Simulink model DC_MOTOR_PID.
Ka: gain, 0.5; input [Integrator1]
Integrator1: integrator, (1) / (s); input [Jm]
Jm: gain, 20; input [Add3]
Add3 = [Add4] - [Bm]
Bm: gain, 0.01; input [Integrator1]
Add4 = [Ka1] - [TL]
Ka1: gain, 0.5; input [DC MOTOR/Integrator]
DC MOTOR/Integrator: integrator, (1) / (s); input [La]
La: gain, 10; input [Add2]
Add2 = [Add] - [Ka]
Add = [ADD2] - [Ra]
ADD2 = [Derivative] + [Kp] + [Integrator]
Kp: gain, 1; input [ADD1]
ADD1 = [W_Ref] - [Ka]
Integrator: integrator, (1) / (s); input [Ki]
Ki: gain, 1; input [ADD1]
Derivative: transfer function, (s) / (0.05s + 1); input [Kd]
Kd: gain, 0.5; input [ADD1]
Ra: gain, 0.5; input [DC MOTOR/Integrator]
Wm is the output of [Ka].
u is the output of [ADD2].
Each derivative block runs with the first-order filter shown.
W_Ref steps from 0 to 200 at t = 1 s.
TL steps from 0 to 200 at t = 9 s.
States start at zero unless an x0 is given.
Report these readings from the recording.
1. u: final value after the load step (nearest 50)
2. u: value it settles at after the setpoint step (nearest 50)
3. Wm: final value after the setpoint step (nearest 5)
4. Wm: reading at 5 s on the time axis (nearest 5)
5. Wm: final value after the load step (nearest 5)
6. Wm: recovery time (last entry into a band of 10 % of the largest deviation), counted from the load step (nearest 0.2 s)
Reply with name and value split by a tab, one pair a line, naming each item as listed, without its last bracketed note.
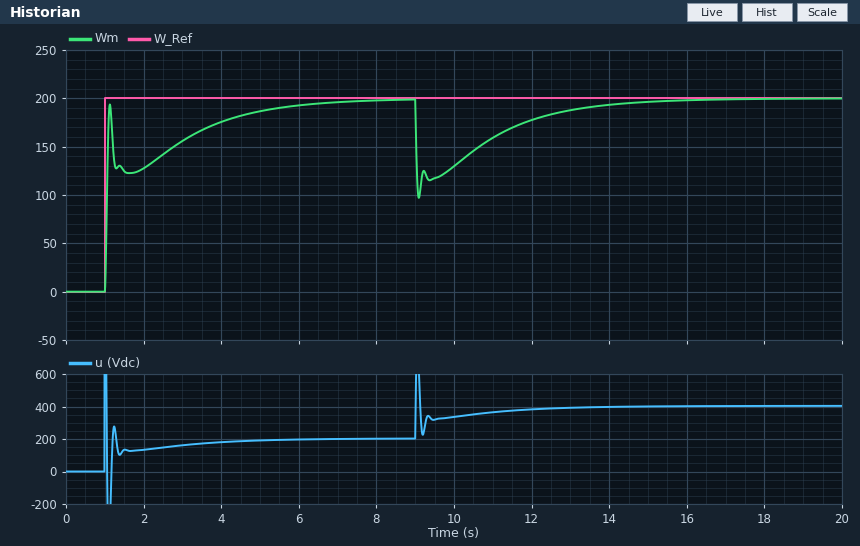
u: final value after the load step	400
u: value it settles at after the setpoint step	200
Wm: final value after the setpoint step	200
Wm: reading at 5 s on the time axis	185
Wm: final value after the load step	200
Wm: recovery time (last entry into a band of 10 % of the largest deviation), counted from the load step	4.4 s
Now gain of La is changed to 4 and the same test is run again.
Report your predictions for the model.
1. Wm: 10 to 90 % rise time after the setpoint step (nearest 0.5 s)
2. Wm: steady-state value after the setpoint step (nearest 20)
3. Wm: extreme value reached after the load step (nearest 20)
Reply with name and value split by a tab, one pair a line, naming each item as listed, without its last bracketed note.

Wm: 10 to 90 % rise time after the setpoint step	3.5 s
Wm: steady-state value after the setpoint step	200
Wm: extreme value reached after the load step	20
